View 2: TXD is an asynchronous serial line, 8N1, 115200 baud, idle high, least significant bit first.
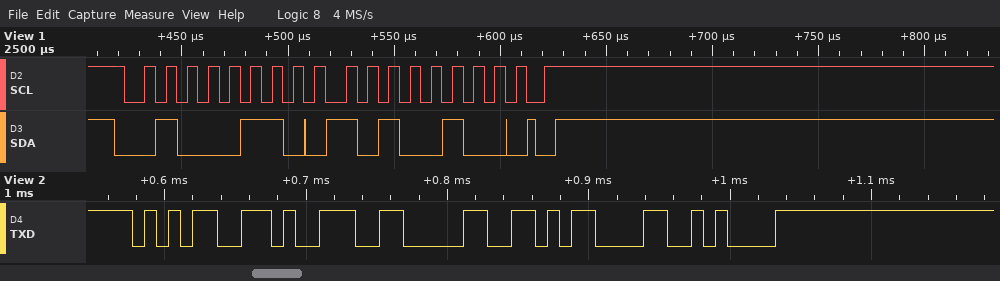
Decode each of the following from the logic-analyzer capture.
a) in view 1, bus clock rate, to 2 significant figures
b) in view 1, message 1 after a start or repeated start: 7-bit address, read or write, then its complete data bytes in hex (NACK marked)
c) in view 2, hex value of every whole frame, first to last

100 kHz
0x23 write: A4
35 39 30 0D 0A
